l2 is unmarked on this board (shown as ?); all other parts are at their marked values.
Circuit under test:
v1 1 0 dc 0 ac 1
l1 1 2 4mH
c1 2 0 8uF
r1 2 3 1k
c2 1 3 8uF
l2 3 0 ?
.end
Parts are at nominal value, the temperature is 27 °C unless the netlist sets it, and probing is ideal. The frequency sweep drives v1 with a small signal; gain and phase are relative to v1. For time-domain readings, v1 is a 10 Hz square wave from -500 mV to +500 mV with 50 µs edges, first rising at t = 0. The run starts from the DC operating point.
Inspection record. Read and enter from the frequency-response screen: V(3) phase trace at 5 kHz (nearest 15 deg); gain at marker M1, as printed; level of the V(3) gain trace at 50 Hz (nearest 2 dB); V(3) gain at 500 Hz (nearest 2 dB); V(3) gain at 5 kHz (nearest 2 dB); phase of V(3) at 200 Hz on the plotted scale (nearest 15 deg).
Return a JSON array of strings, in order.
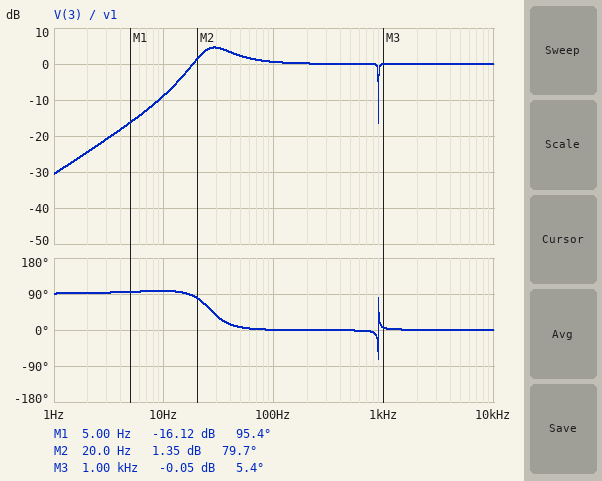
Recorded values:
["0 deg", "-16.12 dB", "2 dB", "0 dB", "0 dB", "0 deg"]
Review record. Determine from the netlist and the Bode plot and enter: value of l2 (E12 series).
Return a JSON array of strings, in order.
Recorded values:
["4.7 H"]
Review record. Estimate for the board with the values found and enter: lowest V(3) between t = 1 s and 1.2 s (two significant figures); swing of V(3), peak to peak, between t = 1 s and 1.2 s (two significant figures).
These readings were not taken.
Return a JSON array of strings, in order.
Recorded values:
["-990 mV", "2.0 V"]
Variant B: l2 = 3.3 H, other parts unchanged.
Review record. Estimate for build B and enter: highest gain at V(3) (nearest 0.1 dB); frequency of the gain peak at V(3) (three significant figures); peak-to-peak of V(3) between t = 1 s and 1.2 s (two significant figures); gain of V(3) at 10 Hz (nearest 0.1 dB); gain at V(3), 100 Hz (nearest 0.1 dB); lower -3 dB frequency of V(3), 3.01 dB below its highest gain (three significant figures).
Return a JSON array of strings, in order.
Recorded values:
["5.6 dB", "33.6 Hz", "2.1 V", "-12.0 dB", "0.8 dB", "25.1 Hz"]
